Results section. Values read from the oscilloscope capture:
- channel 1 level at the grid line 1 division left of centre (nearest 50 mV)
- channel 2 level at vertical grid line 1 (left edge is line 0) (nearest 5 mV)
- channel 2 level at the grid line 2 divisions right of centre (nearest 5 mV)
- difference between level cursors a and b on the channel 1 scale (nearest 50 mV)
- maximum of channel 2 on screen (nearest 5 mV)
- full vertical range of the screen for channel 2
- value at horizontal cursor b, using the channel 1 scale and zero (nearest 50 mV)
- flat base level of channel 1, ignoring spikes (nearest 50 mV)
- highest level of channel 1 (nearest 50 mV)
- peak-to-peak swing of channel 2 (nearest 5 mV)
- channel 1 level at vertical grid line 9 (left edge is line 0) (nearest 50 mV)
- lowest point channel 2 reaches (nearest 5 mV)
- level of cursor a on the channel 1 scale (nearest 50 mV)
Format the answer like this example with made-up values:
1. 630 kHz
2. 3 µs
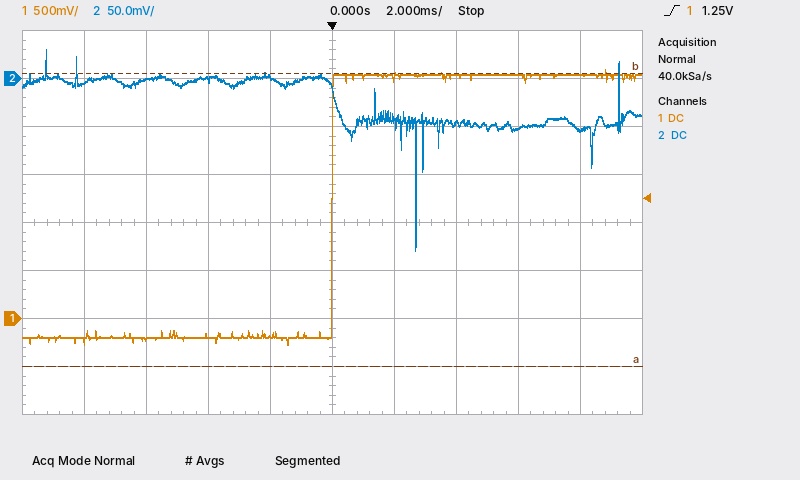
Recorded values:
1. -200 mV
2. -5 mV
3. -45 mV
4. 3.05 V
5. 30 mV
6. 400 mV
7. 2.55 V
8. -200 mV
9. 2.60 V
10. 210 mV
11. 2.55 V
12. -180 mV
13. -500 mV
